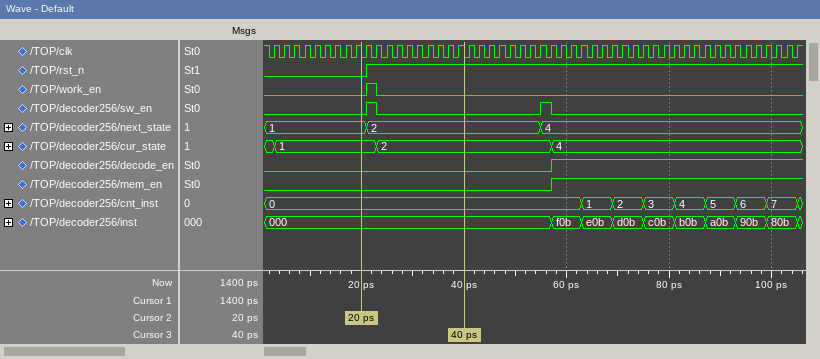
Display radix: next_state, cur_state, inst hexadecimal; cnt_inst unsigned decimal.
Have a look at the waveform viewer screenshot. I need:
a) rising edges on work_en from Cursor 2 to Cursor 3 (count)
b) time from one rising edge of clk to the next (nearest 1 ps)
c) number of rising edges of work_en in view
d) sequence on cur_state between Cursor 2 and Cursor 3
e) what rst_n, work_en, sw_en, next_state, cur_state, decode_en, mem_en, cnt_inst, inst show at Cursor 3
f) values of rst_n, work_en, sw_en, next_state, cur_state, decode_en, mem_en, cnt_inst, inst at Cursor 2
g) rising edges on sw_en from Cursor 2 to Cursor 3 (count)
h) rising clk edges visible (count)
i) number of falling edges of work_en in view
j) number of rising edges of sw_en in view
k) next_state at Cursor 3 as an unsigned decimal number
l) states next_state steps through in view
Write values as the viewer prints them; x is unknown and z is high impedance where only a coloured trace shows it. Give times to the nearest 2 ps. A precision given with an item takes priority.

1
2 ps
1
1, 2
rst_n=1, work_en=0, sw_en=0, next_state=2, cur_state=2, decode_en=0, mem_en=0, cnt_inst=0, inst=000
rst_n=0, work_en=0, sw_en=0, next_state=1, cur_state=1, decode_en=0, mem_en=0, cnt_inst=0, inst=000
1
52
1
2
2
1, 2, 4
